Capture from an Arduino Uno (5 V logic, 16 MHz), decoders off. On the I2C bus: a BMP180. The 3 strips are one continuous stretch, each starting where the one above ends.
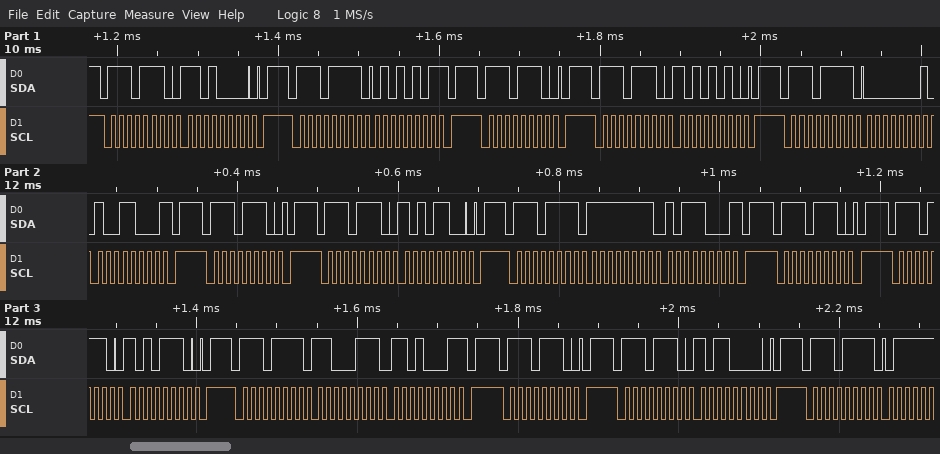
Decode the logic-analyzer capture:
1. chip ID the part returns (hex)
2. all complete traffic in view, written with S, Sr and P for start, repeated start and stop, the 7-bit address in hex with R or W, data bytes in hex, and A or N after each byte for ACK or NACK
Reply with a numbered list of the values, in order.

1. 0x55
2. S 77W A D0 A P S 77R A 55 N P S 77W A P S 77W A AA A P S 77R A 01 A 98 N P S 77W A P S 77W A AC A P S 77R A FF A B8 N P S 77W A P S 77W A AE A P S 77R A C7 A D1 N P S 77W A P S 77W A B0 A P S 77R A
